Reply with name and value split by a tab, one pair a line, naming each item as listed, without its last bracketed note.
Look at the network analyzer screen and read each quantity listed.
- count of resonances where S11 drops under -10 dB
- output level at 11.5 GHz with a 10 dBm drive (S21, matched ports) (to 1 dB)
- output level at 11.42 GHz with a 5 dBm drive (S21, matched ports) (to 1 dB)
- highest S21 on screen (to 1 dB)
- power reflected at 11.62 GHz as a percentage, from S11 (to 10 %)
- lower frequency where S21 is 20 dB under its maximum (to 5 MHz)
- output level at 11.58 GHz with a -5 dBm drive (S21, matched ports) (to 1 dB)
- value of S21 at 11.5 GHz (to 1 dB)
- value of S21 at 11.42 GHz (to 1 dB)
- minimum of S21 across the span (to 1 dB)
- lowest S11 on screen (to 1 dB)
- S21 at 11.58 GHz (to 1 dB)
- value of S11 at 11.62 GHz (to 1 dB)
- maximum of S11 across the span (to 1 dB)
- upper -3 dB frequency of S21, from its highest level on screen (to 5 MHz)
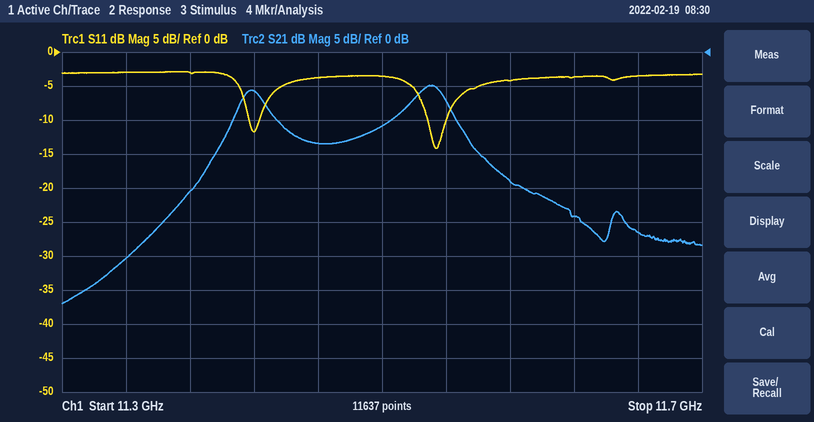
count of resonances where S11 drops under -10 dB	2
output level at 11.5 GHz with a 10 dBm drive (S21, matched ports)	-1 dBm
output level at 11.42 GHz with a 5 dBm drive (S21, matched ports)	-1 dBm
highest S21 on screen	-5 dB
power reflected at 11.62 GHz as a percentage, from S11	40 %
lower frequency where S21 is 20 dB under its maximum	11.365 GHz
output level at 11.58 GHz with a -5 dBm drive (S21, matched ports)	-24 dBm
value of S21 at 11.5 GHz	-11 dB
value of S21 at 11.42 GHz	-6 dB
minimum of S21 across the span	-37 dB
lowest S11 on screen	-14 dB
S21 at 11.58 GHz	-19 dB
value of S11 at 11.62 GHz	-4 dB
maximum of S11 across the span	-3 dB
upper -3 dB frequency of S21, from its highest level on screen	11.540 GHz
